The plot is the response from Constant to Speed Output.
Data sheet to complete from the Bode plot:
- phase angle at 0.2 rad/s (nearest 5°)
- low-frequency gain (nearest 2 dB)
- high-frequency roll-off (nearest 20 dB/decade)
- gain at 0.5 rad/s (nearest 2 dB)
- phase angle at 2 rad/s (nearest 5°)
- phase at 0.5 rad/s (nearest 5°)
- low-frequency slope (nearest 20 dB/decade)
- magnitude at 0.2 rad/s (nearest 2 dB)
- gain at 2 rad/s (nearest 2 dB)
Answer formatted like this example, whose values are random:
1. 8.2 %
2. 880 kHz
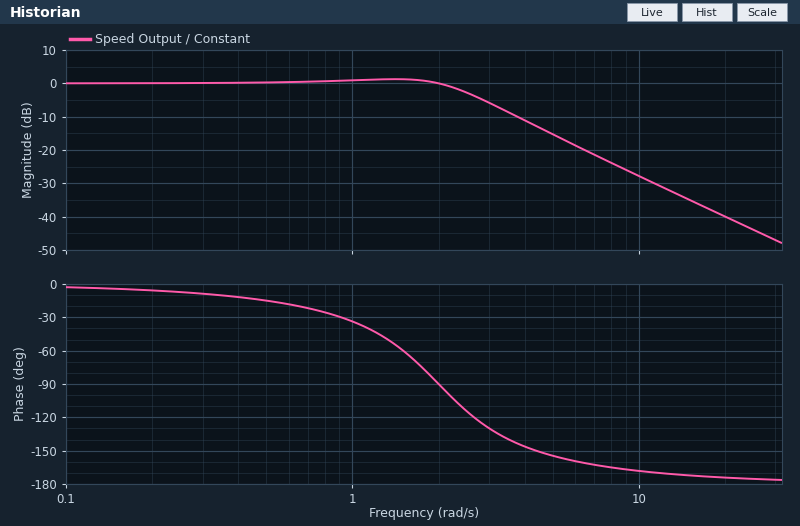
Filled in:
1. -5°
2. 0 dB
3. -40 dB/decade
4. 0 dB
5. -90°
6. -15°
7. 0 dB/decade
8. 0 dB
9. 0 dB
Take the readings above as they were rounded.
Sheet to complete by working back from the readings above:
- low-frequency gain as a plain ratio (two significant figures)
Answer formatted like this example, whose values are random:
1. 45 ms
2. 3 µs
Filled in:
1. 1.0
